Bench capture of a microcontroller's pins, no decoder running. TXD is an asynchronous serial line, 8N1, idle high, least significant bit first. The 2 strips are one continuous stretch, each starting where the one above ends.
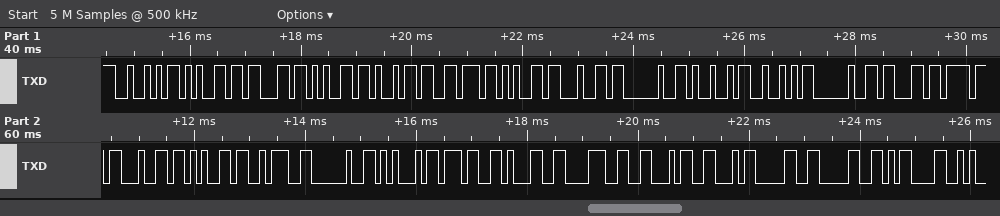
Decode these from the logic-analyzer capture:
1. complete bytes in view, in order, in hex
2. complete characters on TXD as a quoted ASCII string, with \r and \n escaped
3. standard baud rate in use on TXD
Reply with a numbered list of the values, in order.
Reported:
1. 52 65 63 65 69 76 65 64 20 49 52 20 63 6F 64 65 3A 20 45 37 31 38 46 46 30 30 0D
2. "Received IR code: E718FF00\r"
3. 9600 baud
